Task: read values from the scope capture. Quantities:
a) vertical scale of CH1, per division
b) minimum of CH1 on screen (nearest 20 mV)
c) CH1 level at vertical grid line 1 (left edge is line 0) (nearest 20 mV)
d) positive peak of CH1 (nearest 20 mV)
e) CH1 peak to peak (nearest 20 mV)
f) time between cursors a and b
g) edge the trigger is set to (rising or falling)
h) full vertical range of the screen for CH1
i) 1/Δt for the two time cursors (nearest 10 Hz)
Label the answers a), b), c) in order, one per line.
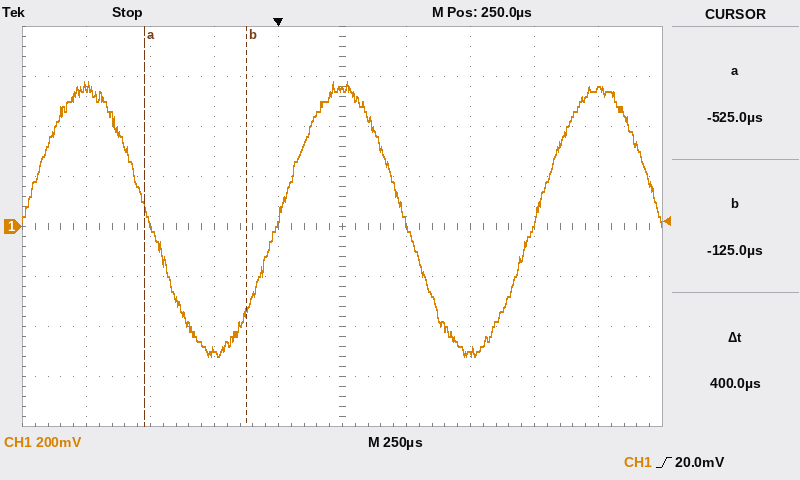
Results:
a) 200 mV
b) -520 mV
c) 560 mV
d) 580 mV
e) 1.10 V
f) 400 µs
g) rising
h) 1.6 V
i) 2.50 kHz
